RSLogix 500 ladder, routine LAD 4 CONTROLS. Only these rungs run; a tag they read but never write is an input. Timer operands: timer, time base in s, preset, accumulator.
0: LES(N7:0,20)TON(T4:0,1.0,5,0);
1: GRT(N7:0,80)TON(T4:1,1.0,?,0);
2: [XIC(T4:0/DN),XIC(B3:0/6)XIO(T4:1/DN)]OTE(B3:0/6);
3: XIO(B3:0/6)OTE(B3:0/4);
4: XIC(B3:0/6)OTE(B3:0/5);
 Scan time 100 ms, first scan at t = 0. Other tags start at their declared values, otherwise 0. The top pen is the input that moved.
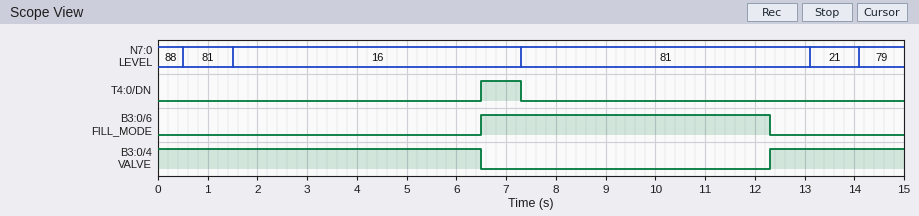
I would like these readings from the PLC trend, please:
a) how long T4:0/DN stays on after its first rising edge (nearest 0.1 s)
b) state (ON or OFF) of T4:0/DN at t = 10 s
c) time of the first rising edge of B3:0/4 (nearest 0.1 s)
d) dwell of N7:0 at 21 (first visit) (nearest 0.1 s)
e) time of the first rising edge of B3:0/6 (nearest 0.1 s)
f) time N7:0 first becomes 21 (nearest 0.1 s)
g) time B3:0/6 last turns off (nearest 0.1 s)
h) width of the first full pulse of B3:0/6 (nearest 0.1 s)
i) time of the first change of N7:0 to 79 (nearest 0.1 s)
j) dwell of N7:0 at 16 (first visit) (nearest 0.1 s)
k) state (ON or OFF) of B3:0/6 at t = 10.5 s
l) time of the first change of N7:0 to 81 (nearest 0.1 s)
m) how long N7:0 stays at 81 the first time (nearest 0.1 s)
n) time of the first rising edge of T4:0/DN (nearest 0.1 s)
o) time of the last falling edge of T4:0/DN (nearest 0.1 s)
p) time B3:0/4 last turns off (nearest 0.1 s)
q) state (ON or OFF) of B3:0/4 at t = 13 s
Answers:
0.8 s
OFF
12.3 s
1.0 s
6.5 s
13.1 s
12.3 s
5.8 s
14.1 s
5.8 s
ON
0.5 s
1.0 s
6.5 s
7.3 s
6.5 s
ON
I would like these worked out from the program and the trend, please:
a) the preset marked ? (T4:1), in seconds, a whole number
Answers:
5 s
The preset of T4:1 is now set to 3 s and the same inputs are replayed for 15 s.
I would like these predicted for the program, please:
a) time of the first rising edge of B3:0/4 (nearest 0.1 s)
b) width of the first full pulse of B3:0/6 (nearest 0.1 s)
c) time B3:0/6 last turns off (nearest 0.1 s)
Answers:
10.3 s
3.8 s
10.3 s
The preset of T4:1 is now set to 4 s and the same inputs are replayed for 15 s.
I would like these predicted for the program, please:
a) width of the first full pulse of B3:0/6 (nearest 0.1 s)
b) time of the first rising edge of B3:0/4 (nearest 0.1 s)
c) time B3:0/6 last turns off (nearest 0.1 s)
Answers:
4.8 s
11.3 s
11.3 s
